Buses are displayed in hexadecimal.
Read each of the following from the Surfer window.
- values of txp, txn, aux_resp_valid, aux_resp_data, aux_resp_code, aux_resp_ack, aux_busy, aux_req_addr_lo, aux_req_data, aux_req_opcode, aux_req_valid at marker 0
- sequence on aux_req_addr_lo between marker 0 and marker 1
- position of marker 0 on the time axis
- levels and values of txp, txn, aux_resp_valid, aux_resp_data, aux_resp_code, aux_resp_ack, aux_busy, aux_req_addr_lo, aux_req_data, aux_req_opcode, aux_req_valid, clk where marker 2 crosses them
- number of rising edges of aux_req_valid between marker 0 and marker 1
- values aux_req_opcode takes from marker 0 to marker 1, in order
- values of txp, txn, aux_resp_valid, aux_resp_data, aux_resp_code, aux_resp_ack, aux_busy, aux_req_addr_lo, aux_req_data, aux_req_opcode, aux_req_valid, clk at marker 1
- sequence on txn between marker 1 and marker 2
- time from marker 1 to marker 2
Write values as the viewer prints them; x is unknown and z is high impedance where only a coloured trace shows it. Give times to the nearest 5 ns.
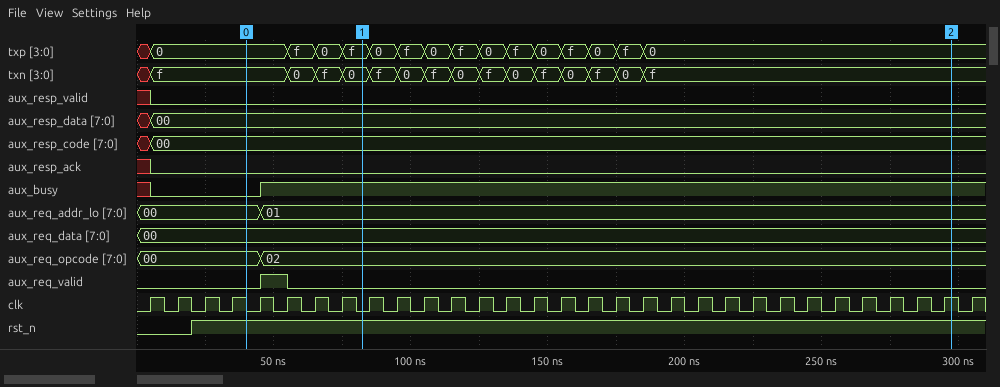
txp=0, txn=f, aux_resp_valid=0, aux_resp_data=00, aux_resp_code=00, aux_resp_ack=0, aux_busy=0, aux_req_addr_lo=00, aux_req_data=00, aux_req_opcode=00, aux_req_valid=0
00, 01
40 ns
txp=0, txn=f, aux_resp_valid=0, aux_resp_data=00, aux_resp_code=00, aux_resp_ack=0, aux_busy=1, aux_req_addr_lo=01, aux_req_data=00, aux_req_opcode=02, aux_req_valid=0, clk=1
1
00, 02
txp=f, txn=0, aux_resp_valid=0, aux_resp_data=00, aux_resp_code=00, aux_resp_ack=0, aux_busy=1, aux_req_addr_lo=01, aux_req_data=00, aux_req_opcode=02, aux_req_valid=0, clk=0
0, f, 0, f, 0, f, 0, f, 0, f, 0, f
215 ns
